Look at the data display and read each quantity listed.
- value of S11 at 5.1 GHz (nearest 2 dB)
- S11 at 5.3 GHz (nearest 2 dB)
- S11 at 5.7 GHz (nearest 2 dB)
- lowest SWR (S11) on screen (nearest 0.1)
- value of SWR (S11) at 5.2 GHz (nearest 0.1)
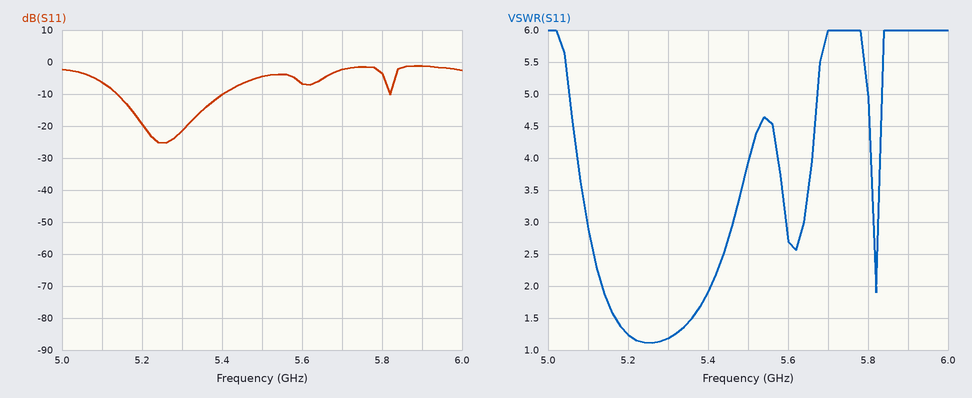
-6 dB
-22 dB
-2 dB
1.1
1.2
